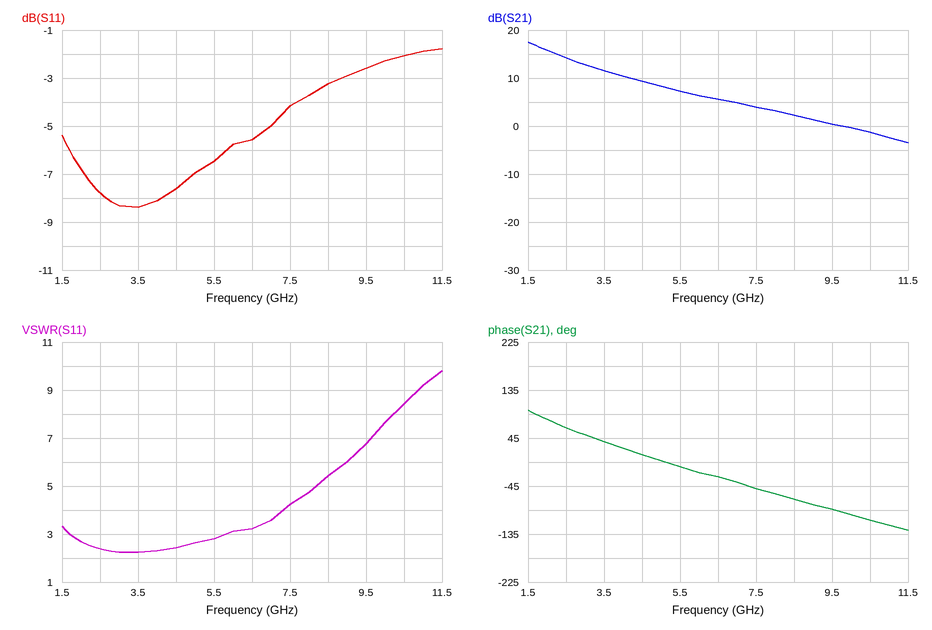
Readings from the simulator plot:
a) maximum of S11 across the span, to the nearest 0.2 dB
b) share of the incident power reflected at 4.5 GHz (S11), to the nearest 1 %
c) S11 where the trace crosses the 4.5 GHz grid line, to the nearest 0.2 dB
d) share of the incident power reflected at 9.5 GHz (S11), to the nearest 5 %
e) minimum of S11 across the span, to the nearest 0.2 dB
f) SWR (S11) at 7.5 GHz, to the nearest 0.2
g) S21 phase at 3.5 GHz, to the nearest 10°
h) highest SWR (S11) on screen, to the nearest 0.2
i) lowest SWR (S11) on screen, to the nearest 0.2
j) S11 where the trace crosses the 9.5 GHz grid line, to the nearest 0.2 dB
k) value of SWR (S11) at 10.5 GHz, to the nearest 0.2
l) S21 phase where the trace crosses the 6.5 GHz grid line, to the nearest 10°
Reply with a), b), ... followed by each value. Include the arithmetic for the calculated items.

a) -1.8 dB
b) 10^(-7.6/10) ≈ 17 %
c) -7.6 dB
d) 10^(-2.6/10) ≈ 55 %
e) -8.4 dB
f) 4.2
g) 40°
h) 9.8
i) 2.2
j) -2.6 dB
k) 8.4
l) -30°
